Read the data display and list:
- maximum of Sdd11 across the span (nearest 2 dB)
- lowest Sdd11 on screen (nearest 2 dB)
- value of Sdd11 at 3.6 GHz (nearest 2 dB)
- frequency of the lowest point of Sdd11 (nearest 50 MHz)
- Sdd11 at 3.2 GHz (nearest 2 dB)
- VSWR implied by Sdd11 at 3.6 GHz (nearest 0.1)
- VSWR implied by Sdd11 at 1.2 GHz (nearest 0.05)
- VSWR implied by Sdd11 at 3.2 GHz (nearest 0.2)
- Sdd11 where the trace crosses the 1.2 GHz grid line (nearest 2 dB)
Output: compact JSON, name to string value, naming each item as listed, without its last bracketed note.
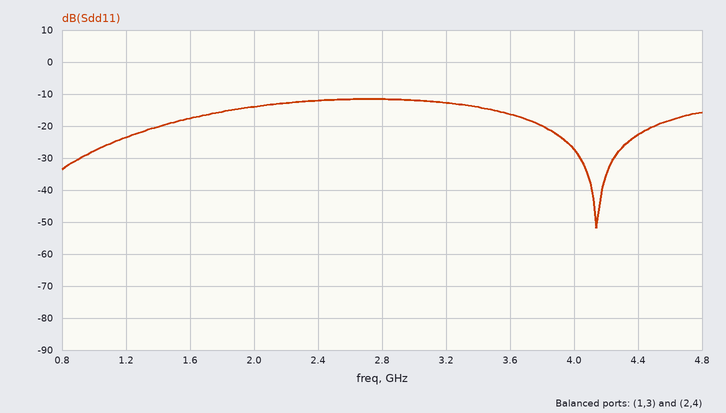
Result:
{"maximum of Sdd11 across the span": "-12 dB", "lowest Sdd11 on screen": "-52 dB", "value of Sdd11 at 3.6 GHz": "-16 dB", "frequency of the lowest point of Sdd11": "4.15 GHz", "Sdd11 at 3.2 GHz": "-12 dB", "VSWR implied by Sdd11 at 3.6 GHz": "1.4", "VSWR implied by Sdd11 at 1.2 GHz": "1.15", "VSWR implied by Sdd11 at 3.2 GHz": "1.6", "Sdd11 where the trace crosses the 1.2 GHz grid line": "-24 dB"}
